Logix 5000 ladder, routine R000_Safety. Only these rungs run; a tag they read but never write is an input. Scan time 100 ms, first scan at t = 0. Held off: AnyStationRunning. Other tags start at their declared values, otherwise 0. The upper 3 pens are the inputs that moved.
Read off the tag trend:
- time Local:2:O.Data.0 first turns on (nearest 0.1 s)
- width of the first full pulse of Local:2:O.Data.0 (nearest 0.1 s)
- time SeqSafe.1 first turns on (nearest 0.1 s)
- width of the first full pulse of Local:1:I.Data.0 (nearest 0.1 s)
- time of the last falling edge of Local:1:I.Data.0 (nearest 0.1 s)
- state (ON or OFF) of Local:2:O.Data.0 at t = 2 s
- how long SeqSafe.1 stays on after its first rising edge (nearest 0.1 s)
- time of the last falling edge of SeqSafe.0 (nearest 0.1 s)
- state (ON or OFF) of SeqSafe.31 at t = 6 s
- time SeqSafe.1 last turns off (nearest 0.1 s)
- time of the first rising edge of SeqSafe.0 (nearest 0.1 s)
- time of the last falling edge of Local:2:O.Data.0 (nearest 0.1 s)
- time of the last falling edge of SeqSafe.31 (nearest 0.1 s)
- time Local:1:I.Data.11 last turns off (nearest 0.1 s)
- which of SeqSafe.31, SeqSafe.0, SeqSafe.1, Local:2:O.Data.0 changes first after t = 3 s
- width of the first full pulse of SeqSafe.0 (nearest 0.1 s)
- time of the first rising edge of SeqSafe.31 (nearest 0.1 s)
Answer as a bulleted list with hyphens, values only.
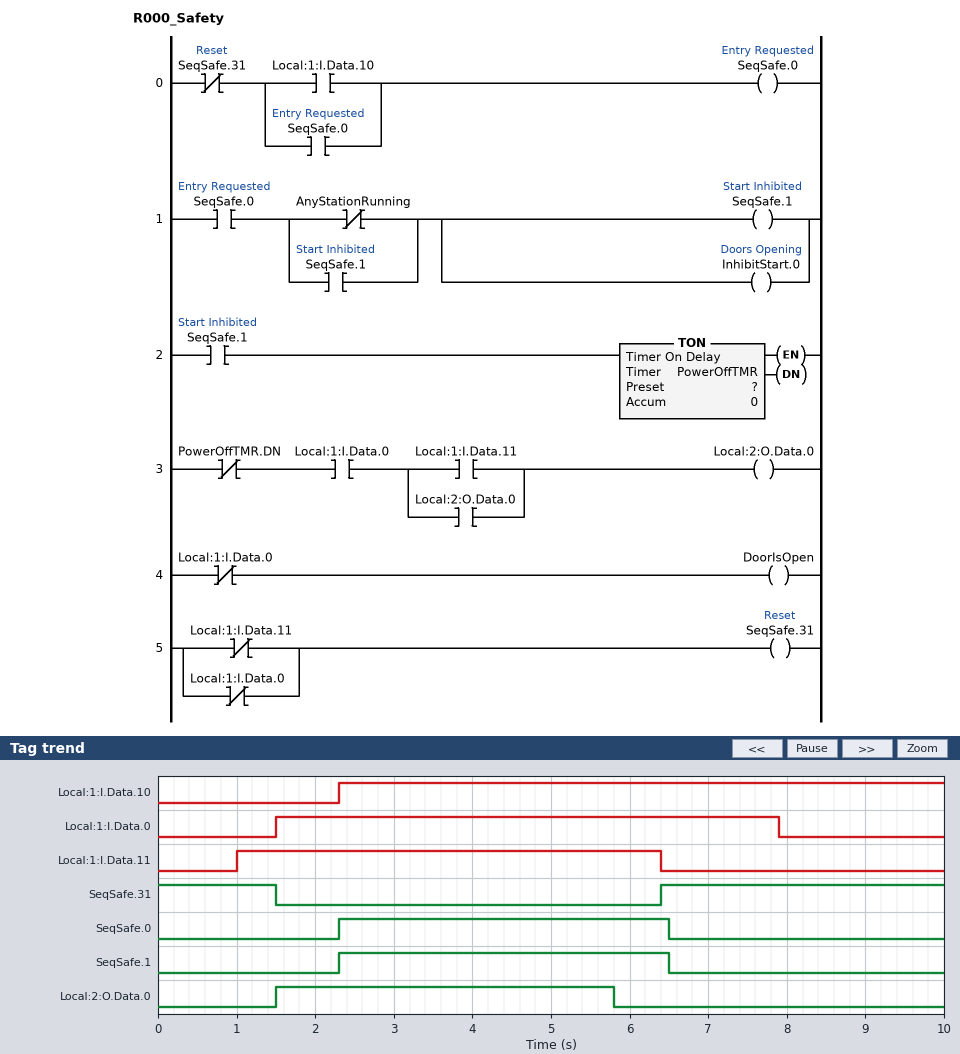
- 1.5 s
- 4.3 s
- 2.3 s
- 6.4 s
- 7.9 s
- ON
- 4.2 s
- 6.5 s
- OFF
- 6.5 s
- 2.3 s
- 5.8 s
- 1.5 s
- 6.4 s
- Local:2:O.Data.0
- 4.2 s
- 6.4 s
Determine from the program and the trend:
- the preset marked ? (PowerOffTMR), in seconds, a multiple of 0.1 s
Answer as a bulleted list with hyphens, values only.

- 3.5 s
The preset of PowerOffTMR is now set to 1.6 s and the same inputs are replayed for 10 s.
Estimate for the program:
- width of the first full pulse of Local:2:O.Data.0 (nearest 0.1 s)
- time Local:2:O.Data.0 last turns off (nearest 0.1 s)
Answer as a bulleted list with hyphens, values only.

- 2.4 s
- 3.9 s
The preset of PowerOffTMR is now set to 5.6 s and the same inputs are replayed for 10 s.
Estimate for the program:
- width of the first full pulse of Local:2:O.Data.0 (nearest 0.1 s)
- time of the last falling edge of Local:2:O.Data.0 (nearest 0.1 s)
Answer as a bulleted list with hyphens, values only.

- 6.4 s
- 7.9 s
